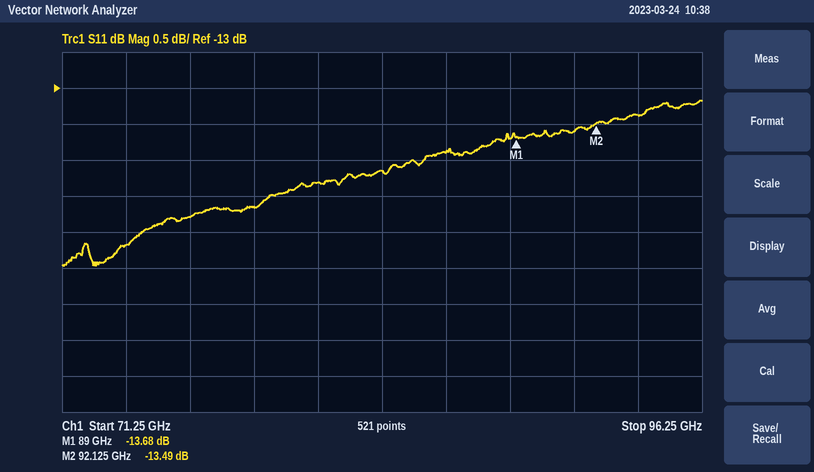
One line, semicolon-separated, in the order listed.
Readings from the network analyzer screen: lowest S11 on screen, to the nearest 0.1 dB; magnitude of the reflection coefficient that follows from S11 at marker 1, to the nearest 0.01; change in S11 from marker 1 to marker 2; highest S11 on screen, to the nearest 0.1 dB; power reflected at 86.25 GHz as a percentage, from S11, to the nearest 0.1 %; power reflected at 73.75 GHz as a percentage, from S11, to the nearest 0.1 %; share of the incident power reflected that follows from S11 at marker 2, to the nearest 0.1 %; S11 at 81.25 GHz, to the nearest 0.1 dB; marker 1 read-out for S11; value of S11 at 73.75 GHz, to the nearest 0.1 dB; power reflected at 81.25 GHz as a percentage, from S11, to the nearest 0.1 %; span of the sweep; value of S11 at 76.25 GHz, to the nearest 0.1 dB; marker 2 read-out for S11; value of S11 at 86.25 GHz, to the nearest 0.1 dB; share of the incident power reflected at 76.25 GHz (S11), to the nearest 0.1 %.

-15.5 dB; 0.21; 0.19 dB; -13.2 dB; 4.1 %; 3.0 %; 4.5 %; -14.3 dB; -13.68 dB; -15.2 dB; 3.7 %; 25 GHz; -14.8 dB; -13.49 dB; -13.9 dB; 3.3 %
